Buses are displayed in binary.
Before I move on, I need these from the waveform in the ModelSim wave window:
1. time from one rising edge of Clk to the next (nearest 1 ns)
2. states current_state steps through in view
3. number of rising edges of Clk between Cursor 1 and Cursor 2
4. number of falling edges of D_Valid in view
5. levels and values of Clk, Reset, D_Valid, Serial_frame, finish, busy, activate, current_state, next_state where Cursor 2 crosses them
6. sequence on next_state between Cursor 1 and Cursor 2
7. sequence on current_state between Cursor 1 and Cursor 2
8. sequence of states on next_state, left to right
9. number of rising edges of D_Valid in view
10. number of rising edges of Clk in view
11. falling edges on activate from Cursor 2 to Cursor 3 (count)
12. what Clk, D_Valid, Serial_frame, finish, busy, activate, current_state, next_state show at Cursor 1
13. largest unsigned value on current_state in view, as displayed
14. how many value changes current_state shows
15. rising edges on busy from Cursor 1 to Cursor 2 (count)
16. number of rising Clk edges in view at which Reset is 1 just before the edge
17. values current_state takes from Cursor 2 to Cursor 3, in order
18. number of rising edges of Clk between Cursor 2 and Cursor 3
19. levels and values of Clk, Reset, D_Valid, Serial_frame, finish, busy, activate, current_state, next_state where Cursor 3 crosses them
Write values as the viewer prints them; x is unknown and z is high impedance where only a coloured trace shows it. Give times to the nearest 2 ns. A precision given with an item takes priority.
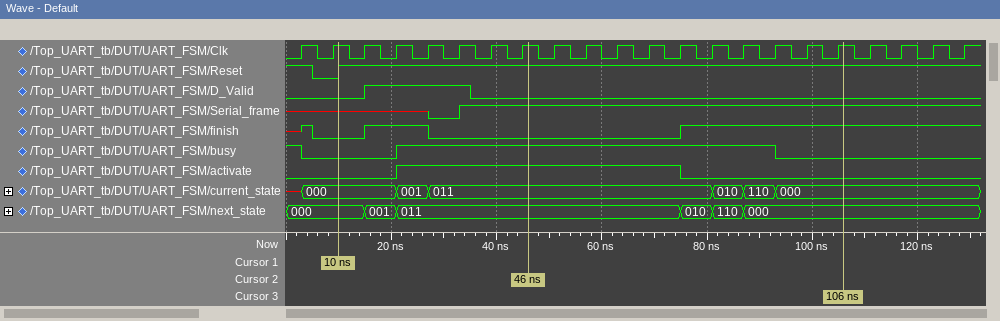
6 ns
x, 000, 001, 011, 010, 110, 000
6
1
Clk=1, Reset=1, D_Valid=0, Serial_frame=1, finish=0, busy=1, activate=1, current_state=011, next_state=011
000, 001, 011
000, 001, 011
000, 001, 011, 010, 110, 000
1
22
1
Clk=1, D_Valid=0, Serial_frame=x, finish=0, busy=0, activate=0, current_state=000, next_state=000
110
6
1
21
011, 010, 110, 000
10
Clk=1, Reset=1, D_Valid=0, Serial_frame=1, finish=1, busy=0, activate=0, current_state=000, next_state=000
